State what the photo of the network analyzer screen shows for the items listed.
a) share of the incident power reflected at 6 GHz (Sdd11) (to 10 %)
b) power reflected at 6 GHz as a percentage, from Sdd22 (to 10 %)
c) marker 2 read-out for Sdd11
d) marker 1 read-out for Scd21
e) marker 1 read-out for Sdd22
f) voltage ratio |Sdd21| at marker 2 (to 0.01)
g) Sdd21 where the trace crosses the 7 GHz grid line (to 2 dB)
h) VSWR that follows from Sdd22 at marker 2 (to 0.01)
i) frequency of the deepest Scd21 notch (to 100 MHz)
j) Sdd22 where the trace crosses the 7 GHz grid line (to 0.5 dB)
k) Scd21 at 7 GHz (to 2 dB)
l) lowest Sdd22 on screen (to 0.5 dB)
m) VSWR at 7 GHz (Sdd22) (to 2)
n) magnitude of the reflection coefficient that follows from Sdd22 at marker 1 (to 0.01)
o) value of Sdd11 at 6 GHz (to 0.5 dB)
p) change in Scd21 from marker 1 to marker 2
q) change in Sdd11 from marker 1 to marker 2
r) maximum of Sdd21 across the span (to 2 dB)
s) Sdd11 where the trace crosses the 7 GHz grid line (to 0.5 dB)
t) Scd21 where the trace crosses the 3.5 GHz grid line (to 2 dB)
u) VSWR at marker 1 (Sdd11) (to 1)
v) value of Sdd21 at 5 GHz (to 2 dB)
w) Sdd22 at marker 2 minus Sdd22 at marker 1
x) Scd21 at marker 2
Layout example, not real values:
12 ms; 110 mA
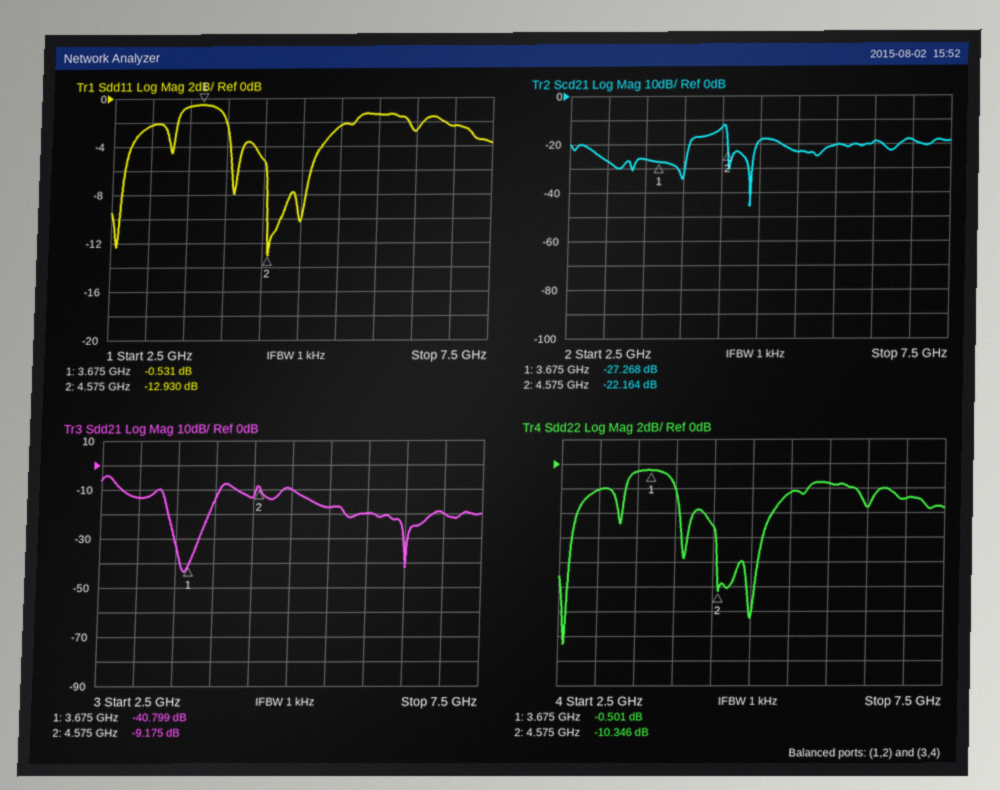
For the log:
70 %; 70 %; -12.930 dB; -27.268 dB; -0.501 dB; 0.35; -20 dB; 1.87; 4.9 GHz; -3.0 dB; -18 dB; -14.5 dB; 6; 0.94; -1.5 dB; 5.104 dB; -12.399 dB; -4 dB; -2.5 dB; -26 dB; 33; -10 dB; -9.845 dB; -22.164 dB
